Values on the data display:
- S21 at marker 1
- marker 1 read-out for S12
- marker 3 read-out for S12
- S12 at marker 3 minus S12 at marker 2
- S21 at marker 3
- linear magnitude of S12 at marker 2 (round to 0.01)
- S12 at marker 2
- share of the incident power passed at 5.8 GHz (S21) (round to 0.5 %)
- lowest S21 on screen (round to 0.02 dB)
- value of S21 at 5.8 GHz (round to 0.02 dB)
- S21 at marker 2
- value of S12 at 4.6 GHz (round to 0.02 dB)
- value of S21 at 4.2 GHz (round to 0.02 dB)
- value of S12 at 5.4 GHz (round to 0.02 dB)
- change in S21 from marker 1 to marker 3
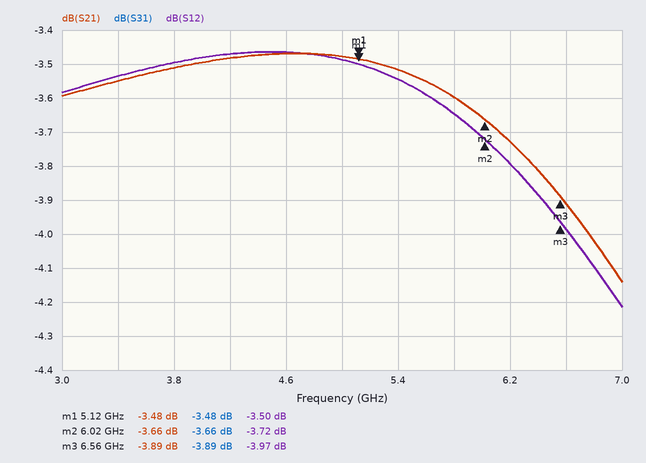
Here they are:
-3.48 dB
-3.50 dB
-3.97 dB
-0.25 dB
-3.89 dB
0.65
-3.72 dB
43.5 %
-4.14 dB
-3.60 dB
-3.66 dB
-3.46 dB
-3.48 dB
-3.54 dB
-0.41 dB
